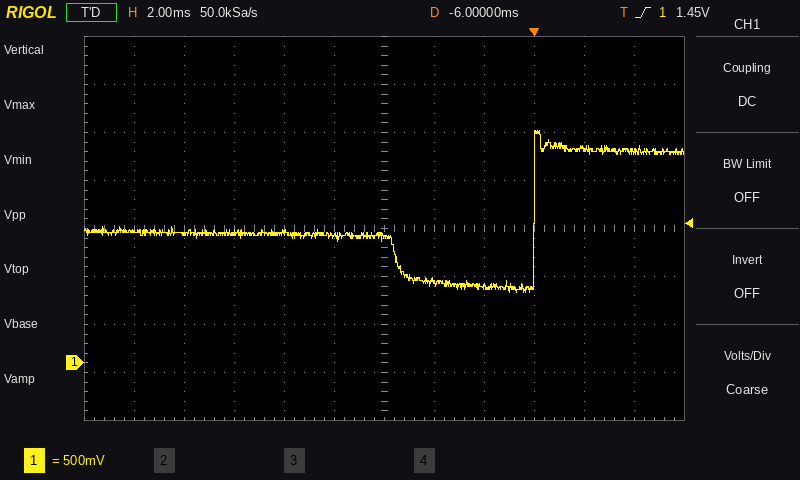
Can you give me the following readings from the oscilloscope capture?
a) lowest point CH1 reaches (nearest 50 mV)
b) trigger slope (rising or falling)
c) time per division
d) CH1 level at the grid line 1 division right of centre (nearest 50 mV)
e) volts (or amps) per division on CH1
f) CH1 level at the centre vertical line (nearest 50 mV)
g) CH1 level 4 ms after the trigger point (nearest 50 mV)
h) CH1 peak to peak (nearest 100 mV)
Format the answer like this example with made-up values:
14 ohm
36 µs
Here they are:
750 mV
rising
2 ms
850 mV
500 mV
1.30 V
2.20 V
1.70 V
